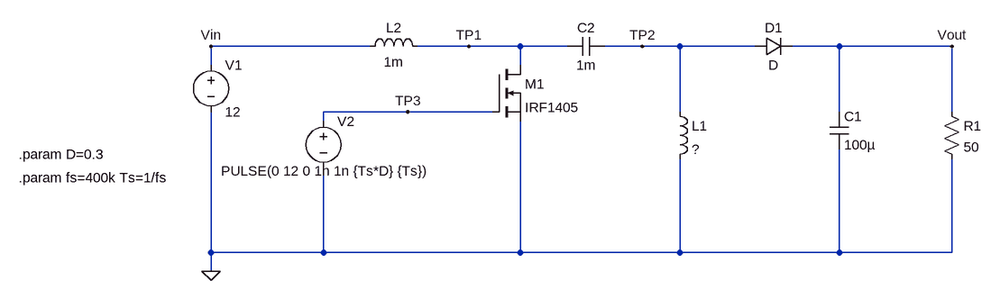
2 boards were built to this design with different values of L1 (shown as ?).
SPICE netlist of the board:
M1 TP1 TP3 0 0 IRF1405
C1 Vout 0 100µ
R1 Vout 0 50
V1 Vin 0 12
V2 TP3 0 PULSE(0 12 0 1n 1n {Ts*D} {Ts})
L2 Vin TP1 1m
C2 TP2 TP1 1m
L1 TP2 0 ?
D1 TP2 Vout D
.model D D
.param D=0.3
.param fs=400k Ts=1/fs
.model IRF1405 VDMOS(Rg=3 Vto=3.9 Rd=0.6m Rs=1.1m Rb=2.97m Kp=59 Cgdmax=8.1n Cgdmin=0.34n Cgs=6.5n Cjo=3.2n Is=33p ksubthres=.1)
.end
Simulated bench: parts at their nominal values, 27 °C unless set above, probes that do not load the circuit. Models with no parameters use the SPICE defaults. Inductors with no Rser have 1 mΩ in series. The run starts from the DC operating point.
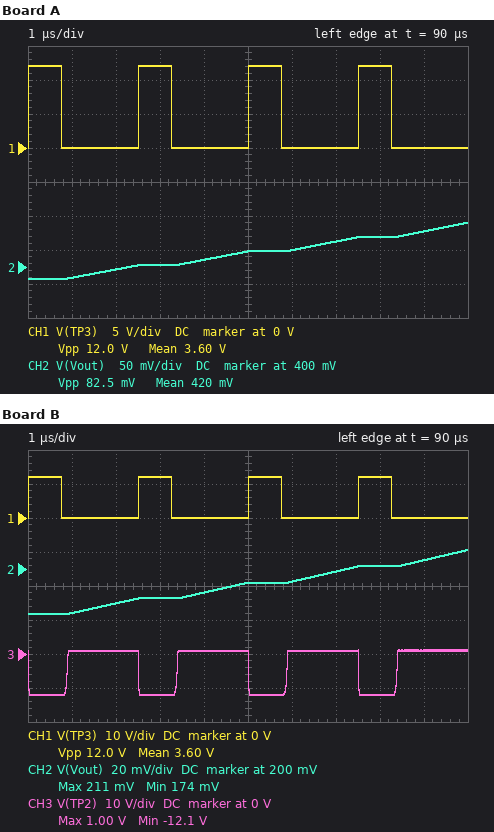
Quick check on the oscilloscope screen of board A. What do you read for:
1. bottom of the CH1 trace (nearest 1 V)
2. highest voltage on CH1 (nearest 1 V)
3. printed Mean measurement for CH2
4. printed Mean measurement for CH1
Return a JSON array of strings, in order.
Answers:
["0 V", "12 V", "420 mV", "3.60 V"]
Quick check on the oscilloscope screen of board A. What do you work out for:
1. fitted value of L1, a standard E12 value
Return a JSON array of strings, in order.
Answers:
["390 µH"]
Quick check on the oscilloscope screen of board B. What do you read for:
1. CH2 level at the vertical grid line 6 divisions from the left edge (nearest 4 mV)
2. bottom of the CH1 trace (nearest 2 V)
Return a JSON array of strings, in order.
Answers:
["192 mV", "0 V"]
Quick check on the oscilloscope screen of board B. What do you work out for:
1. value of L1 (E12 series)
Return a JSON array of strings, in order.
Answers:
["2.2 mH"]
